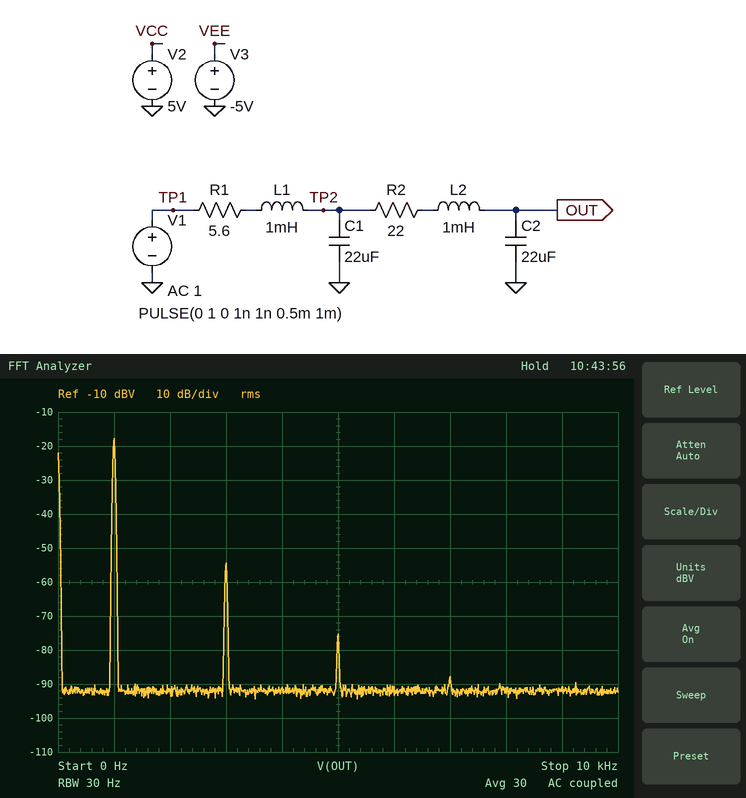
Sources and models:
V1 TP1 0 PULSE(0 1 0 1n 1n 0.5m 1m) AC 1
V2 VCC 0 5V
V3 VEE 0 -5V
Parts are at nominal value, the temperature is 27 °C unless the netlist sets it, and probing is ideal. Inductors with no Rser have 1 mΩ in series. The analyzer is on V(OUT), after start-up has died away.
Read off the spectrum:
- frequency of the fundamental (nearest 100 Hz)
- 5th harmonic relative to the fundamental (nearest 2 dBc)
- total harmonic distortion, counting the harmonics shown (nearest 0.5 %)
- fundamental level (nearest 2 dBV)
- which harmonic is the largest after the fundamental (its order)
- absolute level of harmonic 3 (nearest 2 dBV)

1.0 kHz
-58 dBc
1.5 %
-18 dBV
3
-54 dBV
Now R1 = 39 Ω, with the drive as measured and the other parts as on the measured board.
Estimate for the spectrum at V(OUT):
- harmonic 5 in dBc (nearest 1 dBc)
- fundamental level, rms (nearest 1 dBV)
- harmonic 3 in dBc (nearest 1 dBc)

-47 dBc
-32 dBV
-30 dBc
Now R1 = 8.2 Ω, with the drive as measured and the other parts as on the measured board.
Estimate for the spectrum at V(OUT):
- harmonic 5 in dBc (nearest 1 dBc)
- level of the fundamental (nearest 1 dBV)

-55 dBc
-20 dBV
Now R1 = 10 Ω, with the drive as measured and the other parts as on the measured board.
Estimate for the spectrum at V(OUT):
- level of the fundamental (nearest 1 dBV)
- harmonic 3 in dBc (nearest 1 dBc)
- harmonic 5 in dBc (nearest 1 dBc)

-22 dBV
-34 dBc
-54 dBc
